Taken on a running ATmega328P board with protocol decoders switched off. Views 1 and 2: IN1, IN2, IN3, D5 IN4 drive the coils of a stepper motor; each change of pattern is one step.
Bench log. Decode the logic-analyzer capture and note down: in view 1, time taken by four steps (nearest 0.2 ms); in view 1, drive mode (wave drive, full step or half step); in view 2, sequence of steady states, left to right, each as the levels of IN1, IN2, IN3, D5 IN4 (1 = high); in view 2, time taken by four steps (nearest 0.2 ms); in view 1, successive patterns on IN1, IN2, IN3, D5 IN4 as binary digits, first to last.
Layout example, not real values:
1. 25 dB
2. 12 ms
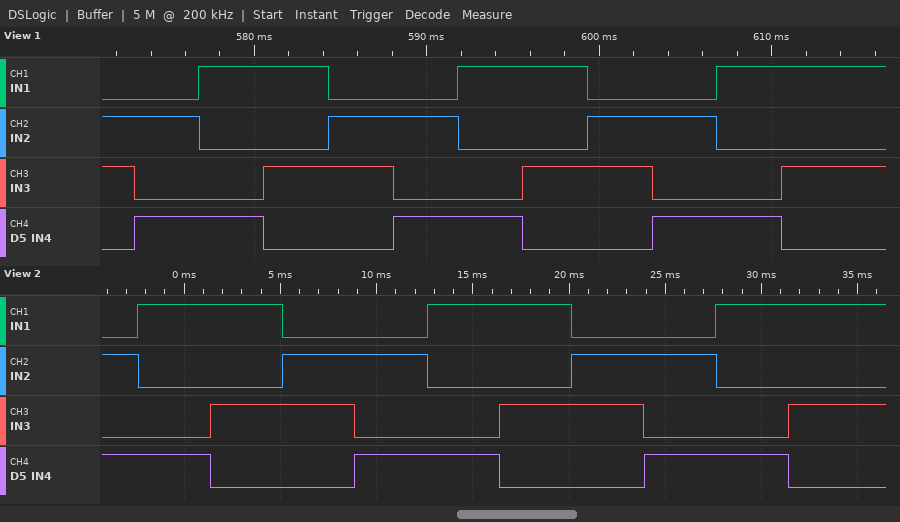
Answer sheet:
1. 15.0 ms
2. full step
3. 0101 1001 1010 0110 0101 1001 1010 0110 0101 1001 1010
4. 15.0 ms
5. 0110 0101 1001 1010 0110 0101 1001 1010 0110 0101 1001 1010
